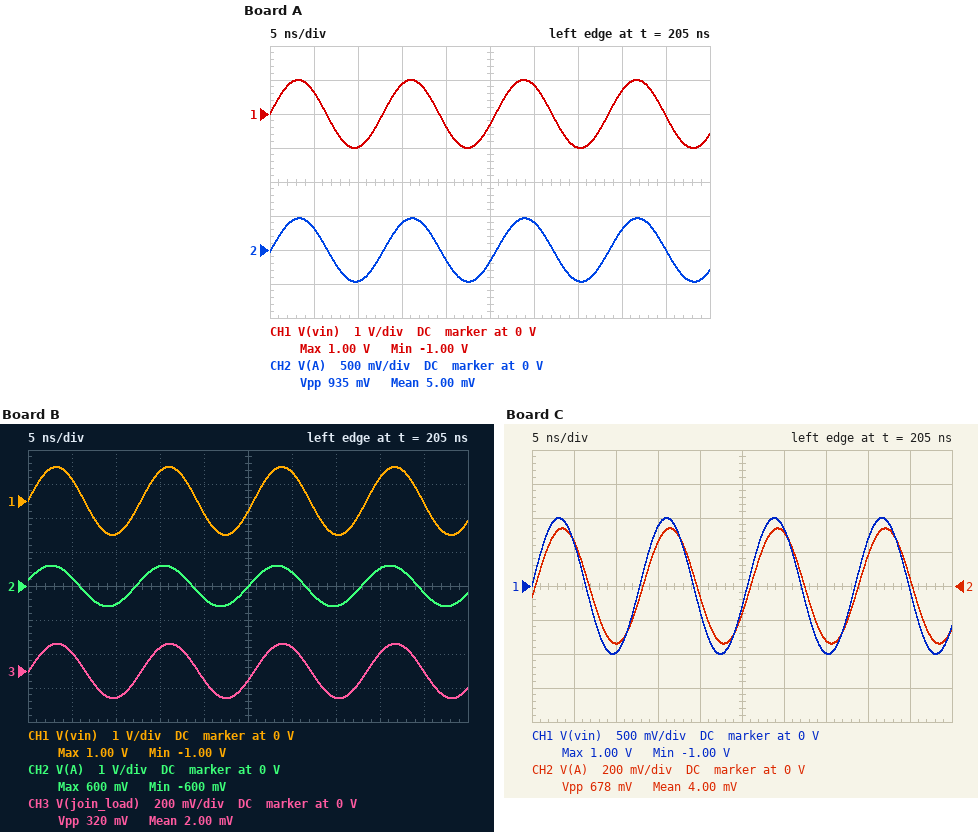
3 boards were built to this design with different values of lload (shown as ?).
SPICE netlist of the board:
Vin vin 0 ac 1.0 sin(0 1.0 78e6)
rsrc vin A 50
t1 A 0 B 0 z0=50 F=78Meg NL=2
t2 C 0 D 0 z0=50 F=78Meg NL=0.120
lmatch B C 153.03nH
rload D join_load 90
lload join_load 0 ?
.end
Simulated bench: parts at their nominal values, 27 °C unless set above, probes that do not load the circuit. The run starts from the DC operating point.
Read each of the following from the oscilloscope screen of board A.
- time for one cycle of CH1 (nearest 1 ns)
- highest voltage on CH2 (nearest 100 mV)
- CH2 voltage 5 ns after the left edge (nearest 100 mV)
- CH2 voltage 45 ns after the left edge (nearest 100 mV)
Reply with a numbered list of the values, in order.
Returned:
1. 13 ns
2. 500 mV
3. 300 mV
4. 0 V
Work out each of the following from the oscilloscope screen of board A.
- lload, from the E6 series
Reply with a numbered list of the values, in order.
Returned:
1. 220 nH
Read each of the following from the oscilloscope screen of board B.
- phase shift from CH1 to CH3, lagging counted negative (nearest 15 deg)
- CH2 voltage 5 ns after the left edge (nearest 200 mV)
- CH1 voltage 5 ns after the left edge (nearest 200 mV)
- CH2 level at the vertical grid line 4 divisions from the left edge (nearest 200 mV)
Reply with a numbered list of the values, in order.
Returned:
1. 0 deg
2. 200 mV
3. 600 mV
4. -400 mV
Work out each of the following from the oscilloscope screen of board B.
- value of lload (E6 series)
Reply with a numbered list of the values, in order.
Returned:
1. 47 nH
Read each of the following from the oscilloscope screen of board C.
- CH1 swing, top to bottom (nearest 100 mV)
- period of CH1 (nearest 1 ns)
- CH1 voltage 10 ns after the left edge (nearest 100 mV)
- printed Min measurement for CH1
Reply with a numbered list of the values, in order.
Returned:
1. 2.0 V
2. 13 ns
3. -1.0 V
4. -1.00 V
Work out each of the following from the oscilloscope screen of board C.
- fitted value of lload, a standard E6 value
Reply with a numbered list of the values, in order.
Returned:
1. 330 nH
